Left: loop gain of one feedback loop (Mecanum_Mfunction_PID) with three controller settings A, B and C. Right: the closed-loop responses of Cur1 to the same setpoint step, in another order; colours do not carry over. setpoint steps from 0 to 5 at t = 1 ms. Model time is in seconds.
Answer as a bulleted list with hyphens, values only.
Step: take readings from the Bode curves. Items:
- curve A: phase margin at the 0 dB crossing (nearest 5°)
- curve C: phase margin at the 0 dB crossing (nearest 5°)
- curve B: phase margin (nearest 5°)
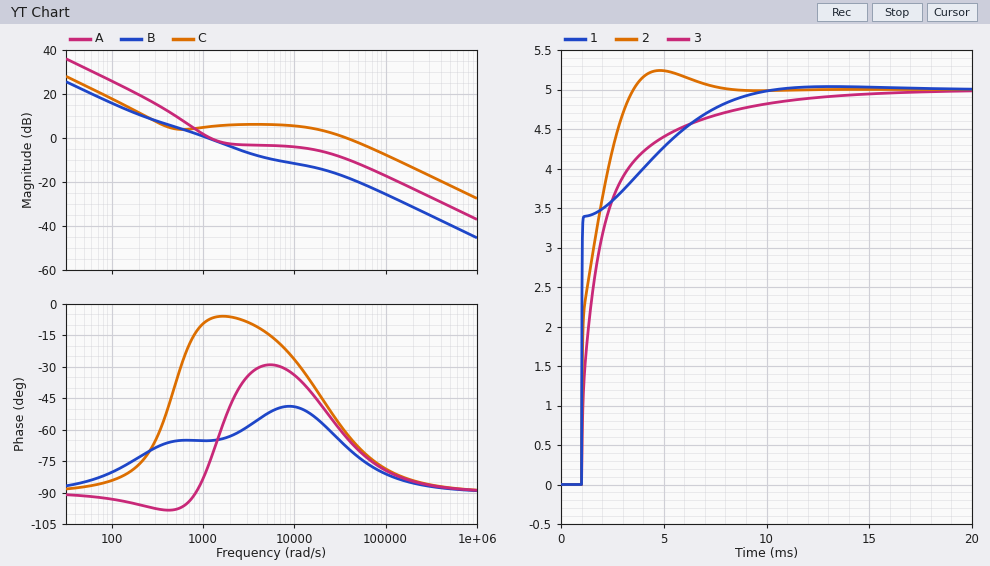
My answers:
- 105°
- 120°
- 115°
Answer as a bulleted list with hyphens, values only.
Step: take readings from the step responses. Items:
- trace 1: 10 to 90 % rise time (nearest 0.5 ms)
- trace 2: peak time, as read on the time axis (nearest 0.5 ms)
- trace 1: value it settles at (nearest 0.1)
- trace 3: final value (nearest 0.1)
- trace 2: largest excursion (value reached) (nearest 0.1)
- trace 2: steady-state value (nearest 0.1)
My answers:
- 5.0 ms
- 5.0 ms
- 5.0
- 5.0
- 5.2
- 5.0
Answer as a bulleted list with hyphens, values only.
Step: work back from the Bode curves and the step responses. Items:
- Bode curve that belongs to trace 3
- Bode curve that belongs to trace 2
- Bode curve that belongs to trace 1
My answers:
- B
- A
- C
